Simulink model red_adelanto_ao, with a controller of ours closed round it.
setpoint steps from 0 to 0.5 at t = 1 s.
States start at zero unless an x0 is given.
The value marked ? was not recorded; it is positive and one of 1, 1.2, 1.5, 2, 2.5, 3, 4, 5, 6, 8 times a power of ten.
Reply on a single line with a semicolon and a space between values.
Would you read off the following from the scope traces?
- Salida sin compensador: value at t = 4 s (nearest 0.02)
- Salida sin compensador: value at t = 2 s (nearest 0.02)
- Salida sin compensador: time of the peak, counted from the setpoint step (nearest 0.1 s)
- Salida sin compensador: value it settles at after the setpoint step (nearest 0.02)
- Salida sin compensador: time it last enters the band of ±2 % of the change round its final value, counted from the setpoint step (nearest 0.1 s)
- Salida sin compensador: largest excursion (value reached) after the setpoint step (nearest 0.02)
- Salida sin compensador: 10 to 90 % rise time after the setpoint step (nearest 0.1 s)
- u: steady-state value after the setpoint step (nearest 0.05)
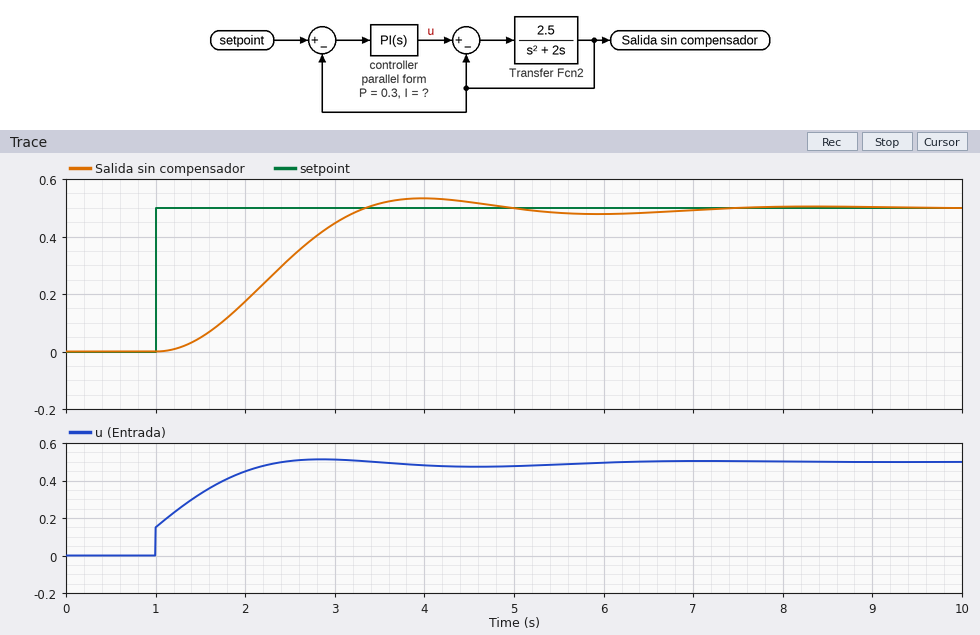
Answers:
0.54; 0.18; 3.0 s; 0.50; 5.9 s; 0.54; 1.5 s; 0.50
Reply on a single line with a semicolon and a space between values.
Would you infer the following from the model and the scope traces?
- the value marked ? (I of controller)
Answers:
0.8
